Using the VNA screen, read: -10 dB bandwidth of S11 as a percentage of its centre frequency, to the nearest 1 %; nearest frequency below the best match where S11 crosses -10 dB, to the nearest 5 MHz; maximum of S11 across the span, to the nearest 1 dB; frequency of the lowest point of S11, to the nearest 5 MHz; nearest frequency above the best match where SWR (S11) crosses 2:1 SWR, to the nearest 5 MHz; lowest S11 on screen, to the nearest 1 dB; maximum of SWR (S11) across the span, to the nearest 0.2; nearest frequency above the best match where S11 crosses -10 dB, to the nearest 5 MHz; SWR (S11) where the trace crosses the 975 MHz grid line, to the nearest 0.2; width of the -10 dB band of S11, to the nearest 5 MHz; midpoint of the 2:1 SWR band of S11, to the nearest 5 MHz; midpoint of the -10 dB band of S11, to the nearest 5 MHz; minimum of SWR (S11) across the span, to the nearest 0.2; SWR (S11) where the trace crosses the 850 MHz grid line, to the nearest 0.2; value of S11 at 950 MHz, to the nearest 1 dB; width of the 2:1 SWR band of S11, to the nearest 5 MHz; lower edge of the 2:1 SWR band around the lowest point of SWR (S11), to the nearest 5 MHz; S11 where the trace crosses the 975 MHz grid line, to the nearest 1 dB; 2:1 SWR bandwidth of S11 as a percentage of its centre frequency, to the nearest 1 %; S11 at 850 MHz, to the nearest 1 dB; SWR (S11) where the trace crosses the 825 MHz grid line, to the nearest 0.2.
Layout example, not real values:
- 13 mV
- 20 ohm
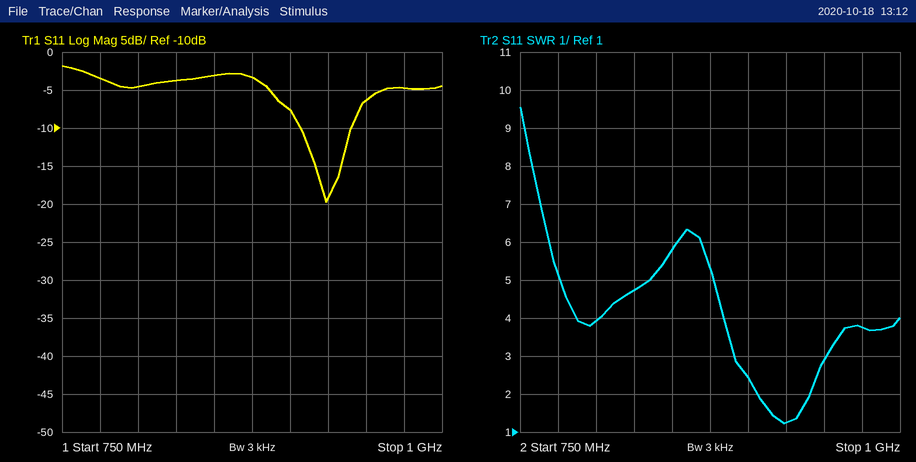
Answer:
- 4 %
- 905 MHz
- -2 dB
- 925 MHz
- 940 MHz
- -20 dB
- 9.6
- 940 MHz
- 3.8
- 35 MHz
- 925 MHz
- 925 MHz
- 1.2
- 5.8
- -6 dB
- 35 MHz
- 905 MHz
- -5 dB
- 4 %
- -3 dB
- 4.8
